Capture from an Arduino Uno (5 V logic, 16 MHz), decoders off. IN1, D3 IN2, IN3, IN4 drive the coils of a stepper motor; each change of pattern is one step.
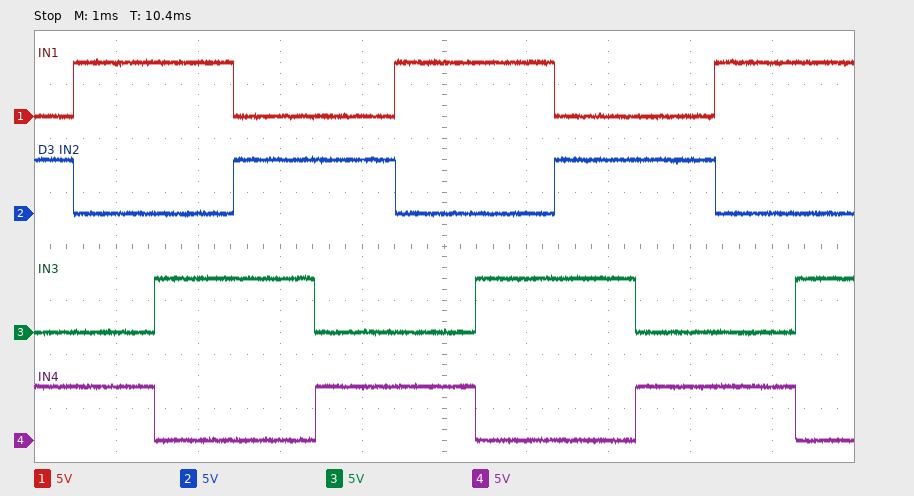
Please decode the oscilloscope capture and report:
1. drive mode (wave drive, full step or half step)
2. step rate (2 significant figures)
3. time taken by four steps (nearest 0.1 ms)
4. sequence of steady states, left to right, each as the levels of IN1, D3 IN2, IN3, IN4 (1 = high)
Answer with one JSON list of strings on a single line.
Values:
["full step", "1000 steps/s", "3.9 ms", "0101 1001 1010 0110 0101 1001 1010 0110 0101 1001 1010"]
